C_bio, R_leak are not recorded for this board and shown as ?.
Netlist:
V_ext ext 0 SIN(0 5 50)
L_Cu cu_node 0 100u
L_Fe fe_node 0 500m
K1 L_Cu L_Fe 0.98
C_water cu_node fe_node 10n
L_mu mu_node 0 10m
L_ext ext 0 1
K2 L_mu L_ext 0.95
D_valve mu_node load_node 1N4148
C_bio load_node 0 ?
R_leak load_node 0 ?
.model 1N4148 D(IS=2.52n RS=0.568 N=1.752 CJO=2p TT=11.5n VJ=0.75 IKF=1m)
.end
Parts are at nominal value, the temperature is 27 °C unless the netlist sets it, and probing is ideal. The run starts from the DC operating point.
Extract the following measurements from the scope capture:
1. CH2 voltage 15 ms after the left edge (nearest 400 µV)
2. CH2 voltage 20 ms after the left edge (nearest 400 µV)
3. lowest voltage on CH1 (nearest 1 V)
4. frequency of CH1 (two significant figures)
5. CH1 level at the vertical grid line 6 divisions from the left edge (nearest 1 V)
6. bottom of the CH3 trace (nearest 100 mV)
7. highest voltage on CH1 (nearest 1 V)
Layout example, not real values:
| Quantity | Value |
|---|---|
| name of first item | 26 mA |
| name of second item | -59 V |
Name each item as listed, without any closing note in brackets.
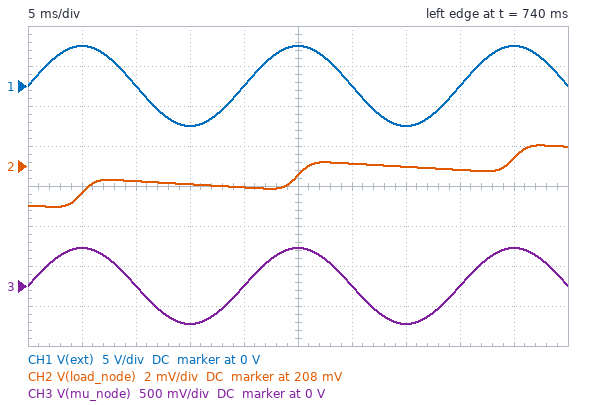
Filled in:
| Quantity | Value |
|---|---|
| CH2 voltage 15 ms after the left edge | 207.2 mV |
| CH2 voltage 20 ms after the left edge | 206.8 mV |
| lowest voltage on CH1 | -5 V |
| frequency of CH1 | 50 Hz |
| CH1 level at the vertical grid line 6 divisions from the left edge | 0 V |
| bottom of the CH3 trace | -500 mV |
| highest voltage on CH1 | 5 V |
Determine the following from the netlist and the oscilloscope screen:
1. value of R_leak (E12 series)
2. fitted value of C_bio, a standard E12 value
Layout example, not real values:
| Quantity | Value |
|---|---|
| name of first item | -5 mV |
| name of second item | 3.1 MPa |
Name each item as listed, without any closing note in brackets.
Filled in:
| Quantity | Value |
|---|---|
| value of R_leak | 4.7 MΩ |
| fitted value of C_bio, a standard E12 value | 1.5 µF |
